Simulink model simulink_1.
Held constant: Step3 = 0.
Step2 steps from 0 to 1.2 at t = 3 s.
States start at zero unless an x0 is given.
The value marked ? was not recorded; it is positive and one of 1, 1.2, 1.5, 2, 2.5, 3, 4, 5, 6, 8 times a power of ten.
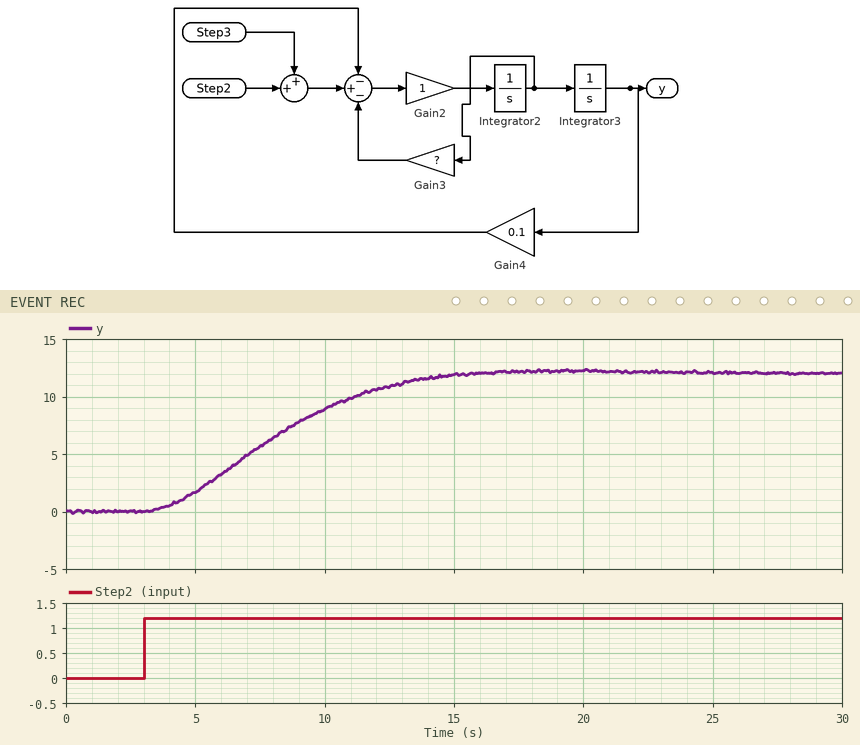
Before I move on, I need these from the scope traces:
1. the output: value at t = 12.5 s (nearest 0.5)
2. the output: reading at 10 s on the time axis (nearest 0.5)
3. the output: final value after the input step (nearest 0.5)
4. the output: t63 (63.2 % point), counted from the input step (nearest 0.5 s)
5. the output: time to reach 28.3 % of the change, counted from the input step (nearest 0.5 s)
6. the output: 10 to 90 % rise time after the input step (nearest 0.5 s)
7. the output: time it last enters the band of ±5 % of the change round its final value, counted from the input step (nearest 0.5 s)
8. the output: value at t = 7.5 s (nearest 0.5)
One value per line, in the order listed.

11.0
9.0
12.0
6.0 s
3.0 s
7.5 s
10.5 s
5.5
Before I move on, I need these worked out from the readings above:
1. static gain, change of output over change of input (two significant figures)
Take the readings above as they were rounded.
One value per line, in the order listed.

10
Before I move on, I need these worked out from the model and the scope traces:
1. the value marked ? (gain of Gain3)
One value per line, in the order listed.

0.5
